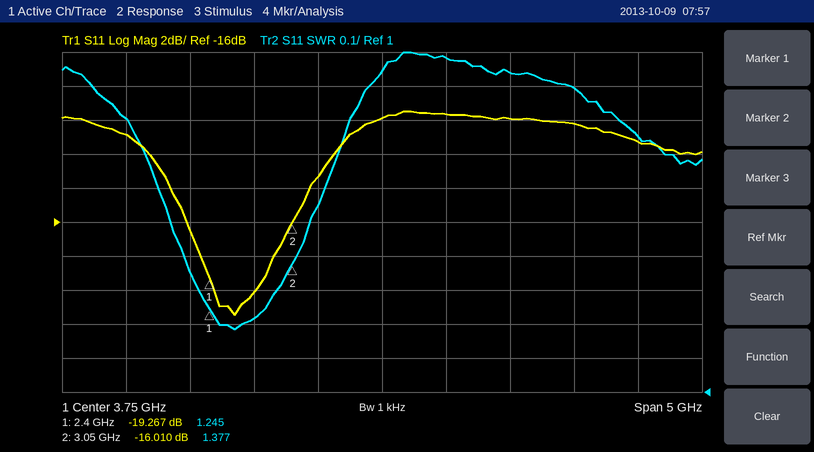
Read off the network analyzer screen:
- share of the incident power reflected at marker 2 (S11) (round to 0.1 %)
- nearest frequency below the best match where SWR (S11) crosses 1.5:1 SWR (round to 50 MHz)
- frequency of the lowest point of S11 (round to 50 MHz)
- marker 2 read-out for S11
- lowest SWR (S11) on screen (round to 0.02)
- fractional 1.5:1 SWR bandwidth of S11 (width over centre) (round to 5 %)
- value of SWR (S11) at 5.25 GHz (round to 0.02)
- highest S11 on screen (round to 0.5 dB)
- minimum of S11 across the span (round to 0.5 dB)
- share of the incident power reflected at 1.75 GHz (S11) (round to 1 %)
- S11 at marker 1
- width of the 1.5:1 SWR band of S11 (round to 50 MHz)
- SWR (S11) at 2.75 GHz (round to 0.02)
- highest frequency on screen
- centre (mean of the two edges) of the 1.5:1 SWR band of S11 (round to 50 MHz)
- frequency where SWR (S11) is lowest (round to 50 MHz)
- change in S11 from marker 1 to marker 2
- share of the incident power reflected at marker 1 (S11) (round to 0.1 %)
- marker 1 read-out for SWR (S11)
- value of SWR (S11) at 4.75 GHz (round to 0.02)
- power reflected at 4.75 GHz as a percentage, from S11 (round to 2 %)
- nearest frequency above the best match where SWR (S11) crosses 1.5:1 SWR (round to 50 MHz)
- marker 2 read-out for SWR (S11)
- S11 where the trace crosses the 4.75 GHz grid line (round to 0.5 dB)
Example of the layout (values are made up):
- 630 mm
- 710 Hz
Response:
- 2.5 %
- 2.10 GHz
- 2.60 GHz
- -16.010 dB
- 1.18
- 40 %
- 1.90
- -9.5 dB
- -21.5 dB
- 8 %
- -19.267 dB
- 1.10 GHz
- 1.22
- 6.25 GHz
- 2.65 GHz
- 2.60 GHz
- 3.257 dB
- 1.2 %
- 1.245
- 1.94
- 10 %
- 3.20 GHz
- 1.377
- -10.0 dB
